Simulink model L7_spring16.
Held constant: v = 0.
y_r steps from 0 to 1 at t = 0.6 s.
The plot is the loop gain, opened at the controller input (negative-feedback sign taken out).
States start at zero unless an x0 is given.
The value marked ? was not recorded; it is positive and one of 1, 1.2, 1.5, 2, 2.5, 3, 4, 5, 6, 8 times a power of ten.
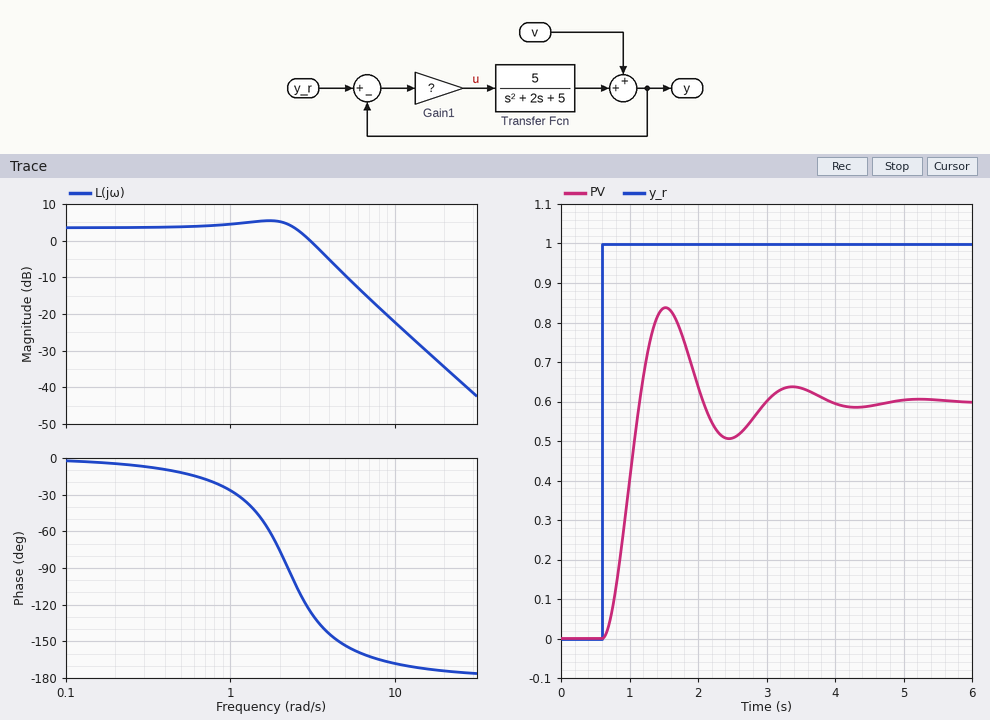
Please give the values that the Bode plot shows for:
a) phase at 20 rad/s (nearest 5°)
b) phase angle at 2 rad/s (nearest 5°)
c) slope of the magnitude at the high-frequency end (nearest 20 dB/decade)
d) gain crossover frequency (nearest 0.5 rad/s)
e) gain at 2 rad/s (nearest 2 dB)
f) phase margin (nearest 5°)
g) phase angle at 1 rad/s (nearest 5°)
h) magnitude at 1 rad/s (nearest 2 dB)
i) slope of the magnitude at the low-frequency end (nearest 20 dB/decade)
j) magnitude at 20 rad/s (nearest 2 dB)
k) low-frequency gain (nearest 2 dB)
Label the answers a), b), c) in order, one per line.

a) -175°
b) -75°
c) -40 dB/decade
d) 3.0 rad/s
e) 6 dB
f) 55°
g) -25°
h) 4 dB
i) 0 dB/decade
j) -34 dB
k) 4 dB
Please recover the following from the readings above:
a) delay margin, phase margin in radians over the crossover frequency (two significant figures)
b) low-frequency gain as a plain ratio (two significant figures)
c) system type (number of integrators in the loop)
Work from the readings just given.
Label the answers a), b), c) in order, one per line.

a) 0.32 s
b) 1.6
c) 0
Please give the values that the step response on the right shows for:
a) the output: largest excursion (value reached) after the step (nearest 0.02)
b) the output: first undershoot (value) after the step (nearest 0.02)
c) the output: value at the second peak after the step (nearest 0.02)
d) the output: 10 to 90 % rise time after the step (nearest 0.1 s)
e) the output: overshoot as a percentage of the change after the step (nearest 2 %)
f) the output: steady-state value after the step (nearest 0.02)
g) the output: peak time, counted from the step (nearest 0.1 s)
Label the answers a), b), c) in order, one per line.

a) 0.84
b) 0.50
c) 0.64
d) 0.4 s
e) 40 %
f) 0.60
g) 0.9 s
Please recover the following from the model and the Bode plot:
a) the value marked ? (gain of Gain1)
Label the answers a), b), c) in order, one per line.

a) 1.5
